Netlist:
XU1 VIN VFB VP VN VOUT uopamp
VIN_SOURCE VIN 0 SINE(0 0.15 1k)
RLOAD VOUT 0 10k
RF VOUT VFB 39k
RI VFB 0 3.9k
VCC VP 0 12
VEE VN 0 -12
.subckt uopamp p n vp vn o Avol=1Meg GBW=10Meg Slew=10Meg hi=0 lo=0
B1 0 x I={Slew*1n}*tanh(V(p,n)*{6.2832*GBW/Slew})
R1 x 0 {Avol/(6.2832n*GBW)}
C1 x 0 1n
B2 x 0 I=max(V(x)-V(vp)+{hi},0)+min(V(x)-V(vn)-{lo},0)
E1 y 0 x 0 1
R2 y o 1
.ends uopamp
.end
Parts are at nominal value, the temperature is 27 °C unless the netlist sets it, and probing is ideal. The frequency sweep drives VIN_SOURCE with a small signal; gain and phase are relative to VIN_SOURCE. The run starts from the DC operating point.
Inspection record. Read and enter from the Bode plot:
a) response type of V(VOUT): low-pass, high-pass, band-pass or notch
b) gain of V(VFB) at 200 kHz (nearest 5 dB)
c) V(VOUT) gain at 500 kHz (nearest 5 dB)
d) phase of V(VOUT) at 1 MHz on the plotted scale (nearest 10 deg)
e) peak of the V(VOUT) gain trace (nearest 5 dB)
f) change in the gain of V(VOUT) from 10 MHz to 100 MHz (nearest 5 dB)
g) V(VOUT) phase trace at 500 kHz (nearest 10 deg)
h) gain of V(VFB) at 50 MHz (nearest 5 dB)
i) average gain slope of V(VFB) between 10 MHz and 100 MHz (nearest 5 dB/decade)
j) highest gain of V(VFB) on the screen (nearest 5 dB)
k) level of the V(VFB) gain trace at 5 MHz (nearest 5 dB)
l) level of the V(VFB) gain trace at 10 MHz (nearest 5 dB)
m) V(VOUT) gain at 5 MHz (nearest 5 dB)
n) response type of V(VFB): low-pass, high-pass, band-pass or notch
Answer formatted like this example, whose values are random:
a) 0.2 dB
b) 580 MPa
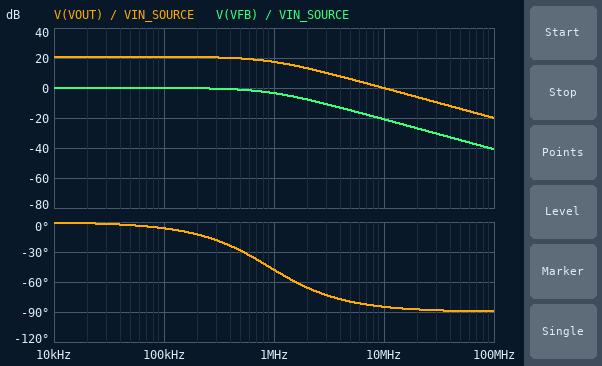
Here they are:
a) low-pass
b) 0 dB
c) 20 dB
d) -50 deg
e) 20 dB
f) -20 dB
g) -30 deg
h) -35 dB
i) -20 dB/decade
j) 0 dB
k) -15 dB
l) -20 dB
m) 5 dB
n) low-pass
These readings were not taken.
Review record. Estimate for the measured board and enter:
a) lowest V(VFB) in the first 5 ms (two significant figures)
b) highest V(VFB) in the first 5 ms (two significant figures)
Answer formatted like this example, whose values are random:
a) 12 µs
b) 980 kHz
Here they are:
a) -150 mV
b) 150 mV
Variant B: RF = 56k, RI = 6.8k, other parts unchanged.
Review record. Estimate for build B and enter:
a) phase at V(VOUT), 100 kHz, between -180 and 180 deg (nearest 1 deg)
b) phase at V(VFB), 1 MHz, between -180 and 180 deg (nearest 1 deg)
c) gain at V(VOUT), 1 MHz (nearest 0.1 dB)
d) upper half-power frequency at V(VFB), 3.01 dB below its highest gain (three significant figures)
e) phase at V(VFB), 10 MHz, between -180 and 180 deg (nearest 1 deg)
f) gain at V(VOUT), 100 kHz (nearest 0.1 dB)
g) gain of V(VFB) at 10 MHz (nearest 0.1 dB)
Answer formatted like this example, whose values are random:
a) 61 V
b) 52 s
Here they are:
a) -5 deg
b) -43 deg
c) 16.6 dB
d) 1.08 MHz
e) -84 deg
f) 19.3 dB
g) -19.4 dB
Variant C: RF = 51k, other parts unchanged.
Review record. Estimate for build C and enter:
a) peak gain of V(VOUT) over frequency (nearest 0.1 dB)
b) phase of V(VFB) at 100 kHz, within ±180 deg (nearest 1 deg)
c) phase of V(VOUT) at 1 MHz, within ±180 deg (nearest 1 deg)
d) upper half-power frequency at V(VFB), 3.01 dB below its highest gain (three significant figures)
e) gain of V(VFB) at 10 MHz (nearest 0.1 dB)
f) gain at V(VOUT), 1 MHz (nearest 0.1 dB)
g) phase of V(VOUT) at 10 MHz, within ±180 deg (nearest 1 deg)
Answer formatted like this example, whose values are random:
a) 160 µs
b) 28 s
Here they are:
a) 23.0 dB
b) -8 deg
c) -55 deg
d) 710 kHz
e) -23.0 dB
f) 18.2 dB
g) -86 deg
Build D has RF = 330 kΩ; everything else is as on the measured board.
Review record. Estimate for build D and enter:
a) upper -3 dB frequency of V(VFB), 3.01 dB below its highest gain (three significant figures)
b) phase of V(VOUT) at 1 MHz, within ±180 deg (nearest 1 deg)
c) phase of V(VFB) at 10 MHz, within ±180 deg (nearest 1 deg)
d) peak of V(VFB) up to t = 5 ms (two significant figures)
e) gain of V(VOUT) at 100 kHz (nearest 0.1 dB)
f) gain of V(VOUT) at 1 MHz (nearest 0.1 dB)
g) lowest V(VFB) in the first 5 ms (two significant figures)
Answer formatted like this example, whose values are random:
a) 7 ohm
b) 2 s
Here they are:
a) 117 kHz
b) -83 deg
c) -89 deg
d) 140 mV
e) 36.3 dB
f) 19.9 dB
g) -140 mV
